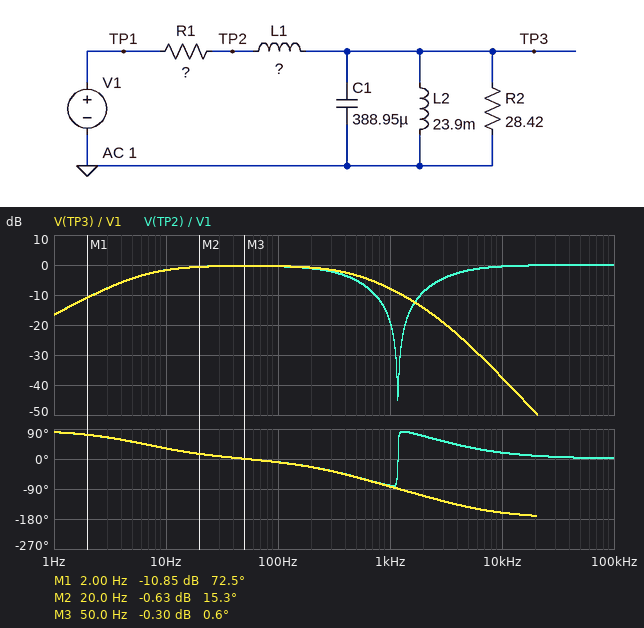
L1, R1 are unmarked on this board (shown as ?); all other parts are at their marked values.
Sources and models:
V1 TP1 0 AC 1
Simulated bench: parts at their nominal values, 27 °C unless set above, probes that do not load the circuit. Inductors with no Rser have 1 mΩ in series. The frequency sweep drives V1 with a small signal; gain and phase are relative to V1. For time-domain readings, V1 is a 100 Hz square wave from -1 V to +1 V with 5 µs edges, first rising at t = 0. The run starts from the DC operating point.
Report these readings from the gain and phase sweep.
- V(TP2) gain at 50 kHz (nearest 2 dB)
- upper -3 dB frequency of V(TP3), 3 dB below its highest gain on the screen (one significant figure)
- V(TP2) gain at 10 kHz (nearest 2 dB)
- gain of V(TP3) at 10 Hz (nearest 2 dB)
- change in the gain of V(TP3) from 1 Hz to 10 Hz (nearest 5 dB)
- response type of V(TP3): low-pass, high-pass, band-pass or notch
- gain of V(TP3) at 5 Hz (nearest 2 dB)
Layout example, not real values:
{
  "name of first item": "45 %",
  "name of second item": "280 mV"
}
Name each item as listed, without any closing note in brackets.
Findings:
{
  "V(TP2) gain at 50 kHz": "0 dB",
  "upper -3 dB frequency of V(TP3), 3 dB below its highest gain on the screen": "500 Hz",
  "V(TP2) gain at 10 kHz": "0 dB",
  "gain of V(TP3) at 10 Hz": "-2 dB",
  "change in the gain of V(TP3) from 1 Hz to 10 Hz": "15 dB",
  "response type of V(TP3): low-pass, high-pass, band-pass or notch": "band-pass",
  "gain of V(TP3) at 5 Hz": "-4 dB"
}
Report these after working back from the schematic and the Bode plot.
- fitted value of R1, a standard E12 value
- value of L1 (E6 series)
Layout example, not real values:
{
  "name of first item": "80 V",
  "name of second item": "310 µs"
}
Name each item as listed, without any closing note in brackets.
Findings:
{
  "fitted value of R1, a standard E12 value": "1 Ω",
  "value of L1": "47 µH"
}
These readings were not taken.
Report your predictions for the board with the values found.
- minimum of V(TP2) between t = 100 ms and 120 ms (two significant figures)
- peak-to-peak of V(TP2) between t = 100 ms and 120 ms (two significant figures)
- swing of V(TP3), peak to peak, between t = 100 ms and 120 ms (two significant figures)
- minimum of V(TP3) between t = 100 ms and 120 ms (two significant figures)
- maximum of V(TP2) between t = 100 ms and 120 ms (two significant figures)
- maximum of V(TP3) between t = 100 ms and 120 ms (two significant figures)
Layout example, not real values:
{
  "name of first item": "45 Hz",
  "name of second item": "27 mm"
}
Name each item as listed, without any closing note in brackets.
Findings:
{
  "minimum of V(TP2) between t = 100 ms and 120 ms": "-1.0 V",
  "peak-to-peak of V(TP2) between t = 100 ms and 120 ms": "2.0 V",
  "swing of V(TP3), peak to peak, between t = 100 ms and 120 ms": "2.0 V",
  "minimum of V(TP3) between t = 100 ms and 120 ms": "-1.0 V",
  "maximum of V(TP2) between t = 100 ms and 120 ms": "1.0 V",
  "maximum of V(TP3) between t = 100 ms and 120 ms": "1.0 V"
}
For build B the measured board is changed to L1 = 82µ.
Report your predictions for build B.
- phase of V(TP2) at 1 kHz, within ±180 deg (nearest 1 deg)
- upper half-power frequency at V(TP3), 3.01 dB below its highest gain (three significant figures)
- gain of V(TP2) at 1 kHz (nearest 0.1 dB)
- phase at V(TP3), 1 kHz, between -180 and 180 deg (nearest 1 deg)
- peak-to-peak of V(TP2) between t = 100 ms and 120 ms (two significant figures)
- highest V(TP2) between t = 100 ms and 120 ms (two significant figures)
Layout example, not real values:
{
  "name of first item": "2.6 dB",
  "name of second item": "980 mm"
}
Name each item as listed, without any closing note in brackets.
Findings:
{
  "phase of V(TP2) at 1 kHz, within ±180 deg": "80 deg",
  "upper half-power frequency at V(TP3), 3.01 dB below its highest gain": "530 Hz",
  "gain of V(TP2) at 1 kHz": "-19.7 dB",
  "phase at V(TP3), 1 kHz, between -180 and 180 deg": "-95 deg",
  "peak-to-peak of V(TP2) between t = 100 ms and 120 ms": "2.1 V",
  "highest V(TP2) between t = 100 ms and 120 ms": "1.1 V"
}
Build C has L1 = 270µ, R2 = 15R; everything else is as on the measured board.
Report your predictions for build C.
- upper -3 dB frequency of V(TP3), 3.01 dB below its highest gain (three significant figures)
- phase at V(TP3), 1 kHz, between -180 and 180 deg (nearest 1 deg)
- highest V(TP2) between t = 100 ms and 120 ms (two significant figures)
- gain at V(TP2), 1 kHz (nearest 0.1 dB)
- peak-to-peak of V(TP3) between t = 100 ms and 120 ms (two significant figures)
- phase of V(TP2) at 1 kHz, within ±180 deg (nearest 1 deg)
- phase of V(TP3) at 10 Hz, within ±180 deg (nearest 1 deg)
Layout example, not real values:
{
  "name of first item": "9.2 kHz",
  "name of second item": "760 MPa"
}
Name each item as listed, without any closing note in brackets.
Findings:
{
  "upper -3 dB frequency of V(TP3), 3.01 dB below its highest gain": "562 Hz",
  "phase at V(TP3), 1 kHz, between -180 and 180 deg": "-140 deg",
  "highest V(TP2) between t = 100 ms and 120 ms": "1.1 V",
  "gain at V(TP2), 1 kHz": "-2.1 dB",
  "peak-to-peak of V(TP3) between t = 100 ms and 120 ms": "2.4 V",
  "phase of V(TP2) at 1 kHz, within ±180 deg": "38 deg",
  "phase of V(TP3) at 10 Hz, within ±180 deg": "31 deg"
}
